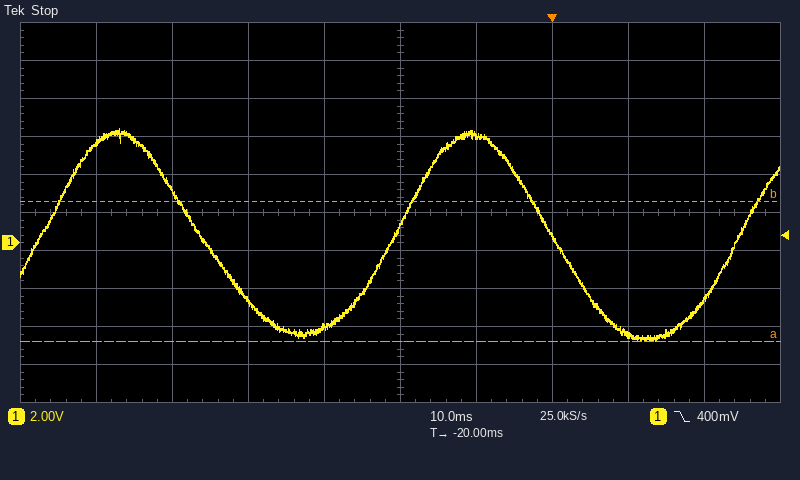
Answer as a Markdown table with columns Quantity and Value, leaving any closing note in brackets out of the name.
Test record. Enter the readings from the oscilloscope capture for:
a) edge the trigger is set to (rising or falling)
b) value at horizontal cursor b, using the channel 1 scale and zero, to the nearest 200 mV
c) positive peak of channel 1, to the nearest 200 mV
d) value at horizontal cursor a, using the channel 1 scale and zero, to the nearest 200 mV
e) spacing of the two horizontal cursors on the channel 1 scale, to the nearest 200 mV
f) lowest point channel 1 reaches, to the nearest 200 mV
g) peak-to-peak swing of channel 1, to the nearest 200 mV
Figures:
| Quantity | Value |
|---|---|
| edge the trigger is set to | falling |
| value at horizontal cursor b, using the channel 1 scale and zero, to the nearest 200 mV | 2.2 V |
| positive peak of channel 1, to the nearest 200 mV | 6.0 V |
| value at horizontal cursor a, using the channel 1 scale and zero, to the nearest 200 mV | -5.2 V |
| spacing of the two horizontal cursors on the channel 1 scale, to the nearest 200 mV | 7.4 V |
| lowest point channel 1 reaches, to the nearest 200 mV | -5.2 V |
| peak-to-peak swing of channel 1, to the nearest 200 mV | 11.2 V |
